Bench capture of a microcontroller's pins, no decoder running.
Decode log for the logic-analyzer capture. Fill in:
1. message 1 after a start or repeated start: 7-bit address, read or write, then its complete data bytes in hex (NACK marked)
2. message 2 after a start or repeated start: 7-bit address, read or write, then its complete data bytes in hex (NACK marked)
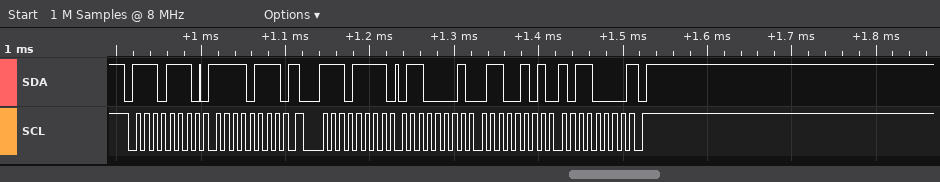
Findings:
0x77 write: F7
0x77 read: 61 65 B0 NACK
